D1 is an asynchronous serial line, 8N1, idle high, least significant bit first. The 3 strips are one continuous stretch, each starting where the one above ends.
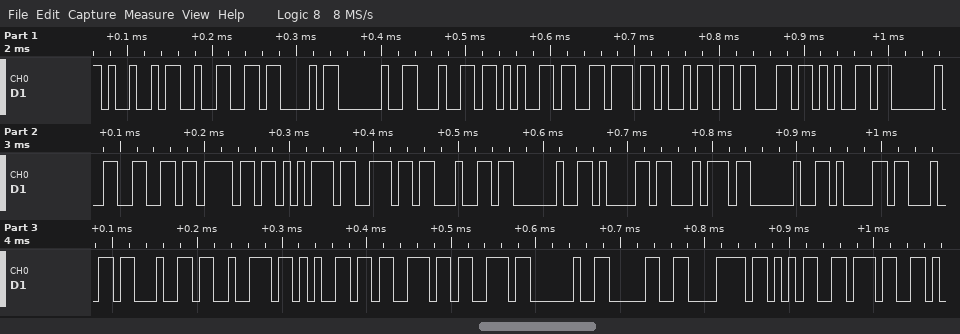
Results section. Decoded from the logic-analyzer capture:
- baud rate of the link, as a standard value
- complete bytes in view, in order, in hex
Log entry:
115200 baud
49 32 43 20 64 65 76 69 63 65 20 66 6F 75 6E 64 20 61 74 20 61 64 64 72 65 73 73 20 30 78 35 37
